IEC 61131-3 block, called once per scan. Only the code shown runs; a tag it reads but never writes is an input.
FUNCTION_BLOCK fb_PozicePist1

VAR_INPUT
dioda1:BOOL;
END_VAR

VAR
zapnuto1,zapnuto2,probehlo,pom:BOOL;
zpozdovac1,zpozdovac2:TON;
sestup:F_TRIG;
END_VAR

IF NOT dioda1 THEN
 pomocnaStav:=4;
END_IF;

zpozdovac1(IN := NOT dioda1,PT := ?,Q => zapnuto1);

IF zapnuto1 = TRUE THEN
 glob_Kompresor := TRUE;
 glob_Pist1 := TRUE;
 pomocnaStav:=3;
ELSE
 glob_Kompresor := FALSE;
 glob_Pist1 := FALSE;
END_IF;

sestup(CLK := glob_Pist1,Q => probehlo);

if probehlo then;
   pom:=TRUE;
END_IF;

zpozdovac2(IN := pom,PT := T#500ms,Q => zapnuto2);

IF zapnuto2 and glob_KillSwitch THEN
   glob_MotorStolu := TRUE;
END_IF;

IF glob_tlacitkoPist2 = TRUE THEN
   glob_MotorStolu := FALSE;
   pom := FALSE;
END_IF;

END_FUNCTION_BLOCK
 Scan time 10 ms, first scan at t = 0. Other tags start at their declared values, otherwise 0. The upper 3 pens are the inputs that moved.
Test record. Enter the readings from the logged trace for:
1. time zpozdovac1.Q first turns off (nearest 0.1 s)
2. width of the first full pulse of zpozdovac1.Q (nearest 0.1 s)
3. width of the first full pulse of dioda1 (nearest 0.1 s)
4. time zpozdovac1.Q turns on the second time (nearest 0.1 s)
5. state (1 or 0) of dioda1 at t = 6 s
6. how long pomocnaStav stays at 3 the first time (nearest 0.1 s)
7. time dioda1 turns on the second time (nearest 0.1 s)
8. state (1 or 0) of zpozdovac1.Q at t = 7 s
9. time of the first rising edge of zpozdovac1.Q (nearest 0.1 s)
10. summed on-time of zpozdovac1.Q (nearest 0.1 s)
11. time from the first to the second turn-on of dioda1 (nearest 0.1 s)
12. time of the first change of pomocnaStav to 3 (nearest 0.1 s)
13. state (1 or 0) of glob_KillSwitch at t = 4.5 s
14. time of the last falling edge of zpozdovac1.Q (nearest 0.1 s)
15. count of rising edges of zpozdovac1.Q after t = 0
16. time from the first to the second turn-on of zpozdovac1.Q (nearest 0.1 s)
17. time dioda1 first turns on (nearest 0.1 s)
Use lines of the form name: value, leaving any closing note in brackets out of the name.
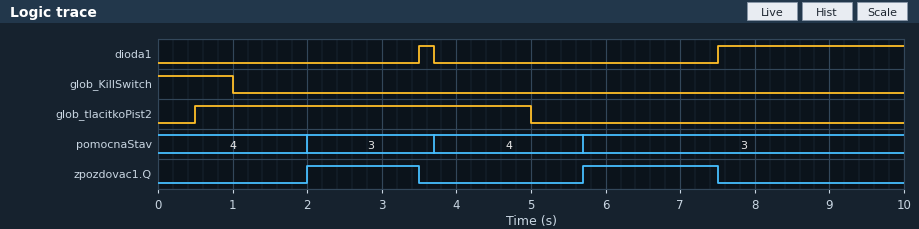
time zpozdovac1.Q first turns off: 3.5 s
width of the first full pulse of zpozdovac1.Q: 1.5 s
width of the first full pulse of dioda1: 0.2 s
time zpozdovac1.Q turns on the second time: 5.7 s
state (1 or 0) of dioda1 at t = 6 s: 0
how long pomocnaStav stays at 3 the first time: 1.7 s
time dioda1 turns on the second time: 7.5 s
state (1 or 0) of zpozdovac1.Q at t = 7 s: 1
time of the first rising edge of zpozdovac1.Q: 2.0 s
summed on-time of zpozdovac1.Q: 3.3 s
time from the first to the second turn-on of dioda1: 4.0 s
time of the first change of pomocnaStav to 3: 2.0 s
state (1 or 0) of glob_KillSwitch at t = 4.5 s: 0
time of the last falling edge of zpozdovac1.Q: 7.5 s
count of rising edges of zpozdovac1.Q after t = 0: 2
time from the first to the second turn-on of zpozdovac1.Q: 3.7 s
time dioda1 first turns on: 3.5 s
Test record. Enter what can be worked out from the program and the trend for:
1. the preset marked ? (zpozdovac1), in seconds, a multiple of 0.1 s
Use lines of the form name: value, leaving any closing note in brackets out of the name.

the preset marked ? (zpozdovac1), in seconds, a multiple of 0.1 s: 2.0 s
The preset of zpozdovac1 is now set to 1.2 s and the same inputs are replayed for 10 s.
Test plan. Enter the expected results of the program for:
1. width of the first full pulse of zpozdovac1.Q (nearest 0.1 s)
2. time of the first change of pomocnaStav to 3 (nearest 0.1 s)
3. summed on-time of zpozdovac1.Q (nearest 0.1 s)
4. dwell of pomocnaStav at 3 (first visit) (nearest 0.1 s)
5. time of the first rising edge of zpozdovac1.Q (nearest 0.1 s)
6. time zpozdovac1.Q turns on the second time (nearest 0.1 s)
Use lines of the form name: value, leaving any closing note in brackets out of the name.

width of the first full pulse of zpozdovac1.Q: 2.3 s
time of the first change of pomocnaStav to 3: 1.2 s
summed on-time of zpozdovac1.Q: 4.9 s
dwell of pomocnaStav at 3 (first visit): 2.5 s
time of the first rising edge of zpozdovac1.Q: 1.2 s
time zpozdovac1.Q turns on the second time: 4.9 s
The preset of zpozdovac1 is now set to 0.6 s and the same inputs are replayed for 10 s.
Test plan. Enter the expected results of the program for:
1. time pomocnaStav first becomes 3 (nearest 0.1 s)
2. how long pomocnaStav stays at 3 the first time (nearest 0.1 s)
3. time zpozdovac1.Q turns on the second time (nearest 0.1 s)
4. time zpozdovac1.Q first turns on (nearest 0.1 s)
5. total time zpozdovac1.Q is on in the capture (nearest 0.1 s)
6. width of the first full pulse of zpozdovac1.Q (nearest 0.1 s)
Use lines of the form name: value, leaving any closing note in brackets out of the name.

time pomocnaStav first becomes 3: 0.6 s
how long pomocnaStav stays at 3 the first time: 3.1 s
time zpozdovac1.Q turns on the second time: 4.3 s
time zpozdovac1.Q first turns on: 0.6 s
total time zpozdovac1.Q is on in the capture: 6.1 s
width of the first full pulse of zpozdovac1.Q: 2.9 s
